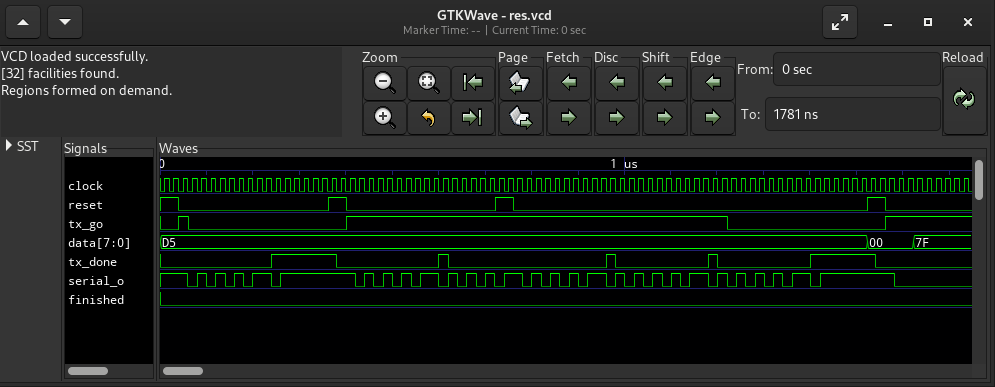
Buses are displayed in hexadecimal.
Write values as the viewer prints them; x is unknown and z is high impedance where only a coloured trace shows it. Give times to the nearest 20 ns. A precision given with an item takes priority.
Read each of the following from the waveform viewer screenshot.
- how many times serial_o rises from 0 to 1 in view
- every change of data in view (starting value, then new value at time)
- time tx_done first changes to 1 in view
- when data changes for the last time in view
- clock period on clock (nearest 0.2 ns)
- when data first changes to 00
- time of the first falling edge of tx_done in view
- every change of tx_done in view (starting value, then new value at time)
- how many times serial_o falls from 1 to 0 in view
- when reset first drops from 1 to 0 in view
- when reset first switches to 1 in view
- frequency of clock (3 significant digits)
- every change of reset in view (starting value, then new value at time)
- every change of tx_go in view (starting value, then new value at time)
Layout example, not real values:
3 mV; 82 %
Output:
28; D5, 00 at 1520 ns, 7F at 1620 ns; 240 ns; 1620 ns; 20 ns; 1520 ns; 380 ns; 0, 1 at 240 ns, 0 at 380 ns, 1 at 600 ns, 0 at 620 ns, 1 at 960 ns, 0 at 980 ns, 1 at 1180 ns, 0 at 1200 ns, 1 at 1400 ns, 0 at 1540 ns; 29; 40 ns; 360 ns; 50.0 MHz; 1, 0 at 40 ns, 1 at 360 ns, 0 at 400 ns, 1 at 720 ns, 0 at 760 ns, 1 at 1520 ns, 0 at 1560 ns; 0, 1 at 40 ns, 0 at 60 ns, 1 at 400 ns, 0 at 1220 ns, 1 at 1560 ns
